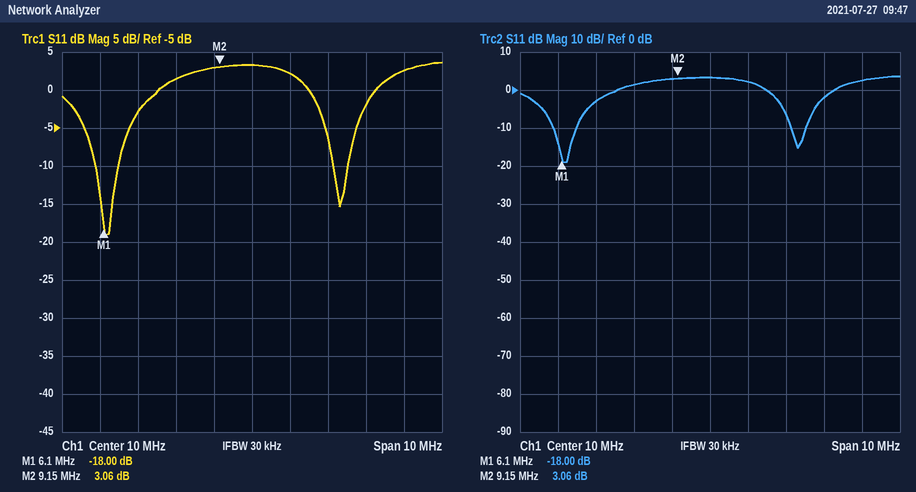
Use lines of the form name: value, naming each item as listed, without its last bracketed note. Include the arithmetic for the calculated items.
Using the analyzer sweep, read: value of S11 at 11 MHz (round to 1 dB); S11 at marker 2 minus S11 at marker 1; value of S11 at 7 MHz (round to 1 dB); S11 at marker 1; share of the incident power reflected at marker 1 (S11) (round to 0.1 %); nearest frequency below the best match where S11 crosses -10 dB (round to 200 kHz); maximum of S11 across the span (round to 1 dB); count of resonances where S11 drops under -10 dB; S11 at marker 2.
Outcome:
value of S11 at 11 MHz: 2 dB
S11 at marker 2 minus S11 at marker 1: 3.06 − (-18) = 21.06 dB
value of S11 at 7 MHz: -3 dB
S11 at marker 1: -18.00 dB
share of the incident power reflected at marker 1 (S11): 10^(-18/10) ≈ 1.6 %
nearest frequency below the best match where S11 crosses -10 dB: 5.8 MHz
maximum of S11 across the span: 4 dB
count of resonances where S11 drops under -10 dB: 2
S11 at marker 2: 3.06 dB
